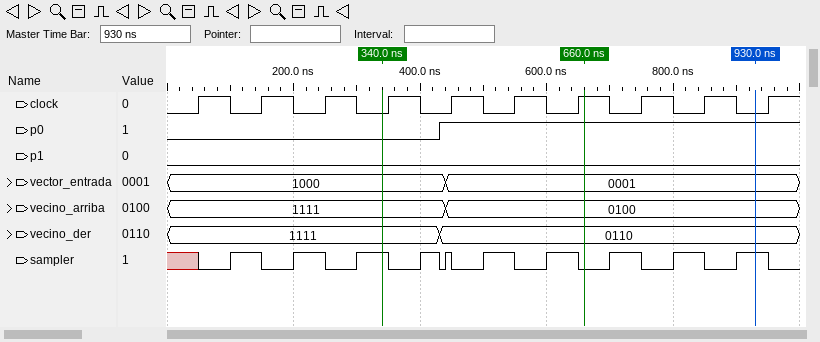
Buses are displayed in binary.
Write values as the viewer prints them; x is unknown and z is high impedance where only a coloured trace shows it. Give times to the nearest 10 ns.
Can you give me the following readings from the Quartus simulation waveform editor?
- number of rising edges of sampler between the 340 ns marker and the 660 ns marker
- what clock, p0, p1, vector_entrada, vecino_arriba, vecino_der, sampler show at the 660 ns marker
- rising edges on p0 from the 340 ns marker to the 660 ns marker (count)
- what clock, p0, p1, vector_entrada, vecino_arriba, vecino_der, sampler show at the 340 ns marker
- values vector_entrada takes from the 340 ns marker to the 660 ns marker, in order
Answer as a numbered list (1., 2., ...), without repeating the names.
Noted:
1. 4
2. clock=1, p0=1, p1=0, vector_entrada=0001, vecino_arriba=0100, vecino_der=0110, sampler=0
3. 1
4. clock=0, p0=0, p1=0, vector_entrada=1000, vecino_arriba=1111, vecino_der=1111, sampler=1
5. 1000, 0001
